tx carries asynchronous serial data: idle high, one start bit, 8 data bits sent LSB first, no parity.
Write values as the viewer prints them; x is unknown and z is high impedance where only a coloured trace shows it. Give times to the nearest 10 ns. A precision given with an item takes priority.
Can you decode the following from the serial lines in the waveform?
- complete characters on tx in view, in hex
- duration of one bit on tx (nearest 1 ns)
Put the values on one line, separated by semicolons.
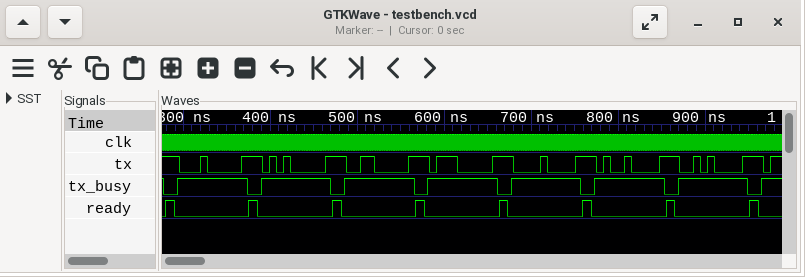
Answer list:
04, 05, 06, 07, 08, 09, 0A; 8 ns
